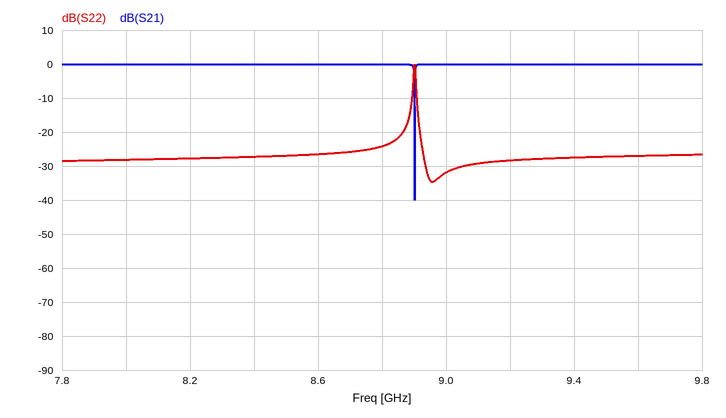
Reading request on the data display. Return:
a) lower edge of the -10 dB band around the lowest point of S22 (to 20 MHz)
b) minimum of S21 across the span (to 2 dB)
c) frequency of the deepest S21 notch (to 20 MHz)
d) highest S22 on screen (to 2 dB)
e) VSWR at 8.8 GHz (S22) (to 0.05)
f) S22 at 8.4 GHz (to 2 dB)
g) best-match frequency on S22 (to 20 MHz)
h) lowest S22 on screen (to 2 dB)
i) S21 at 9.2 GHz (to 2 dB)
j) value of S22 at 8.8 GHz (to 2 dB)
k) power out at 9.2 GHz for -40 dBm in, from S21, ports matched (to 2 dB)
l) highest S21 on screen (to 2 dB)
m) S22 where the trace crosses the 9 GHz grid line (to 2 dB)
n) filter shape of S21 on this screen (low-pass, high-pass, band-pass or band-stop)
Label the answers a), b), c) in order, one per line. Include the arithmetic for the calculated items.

a) 8.90 GHz
b) -40 dB
c) 8.90 GHz
d) 0 dB
e) |Γ| = 10^(-24/20) = 0.0631; VSWR = (1 + 0.0631)/(1 − 0.0631) ≈ 1.13, so 1.15 to the nearest 0.05
f) -28 dB
g) 8.96 GHz
h) -34 dB
i) 0 dB
j) -24 dB
k) -40 dBm + (0 dB) = -40 dBm
l) 0 dB
m) -32 dB
n) band-stop
